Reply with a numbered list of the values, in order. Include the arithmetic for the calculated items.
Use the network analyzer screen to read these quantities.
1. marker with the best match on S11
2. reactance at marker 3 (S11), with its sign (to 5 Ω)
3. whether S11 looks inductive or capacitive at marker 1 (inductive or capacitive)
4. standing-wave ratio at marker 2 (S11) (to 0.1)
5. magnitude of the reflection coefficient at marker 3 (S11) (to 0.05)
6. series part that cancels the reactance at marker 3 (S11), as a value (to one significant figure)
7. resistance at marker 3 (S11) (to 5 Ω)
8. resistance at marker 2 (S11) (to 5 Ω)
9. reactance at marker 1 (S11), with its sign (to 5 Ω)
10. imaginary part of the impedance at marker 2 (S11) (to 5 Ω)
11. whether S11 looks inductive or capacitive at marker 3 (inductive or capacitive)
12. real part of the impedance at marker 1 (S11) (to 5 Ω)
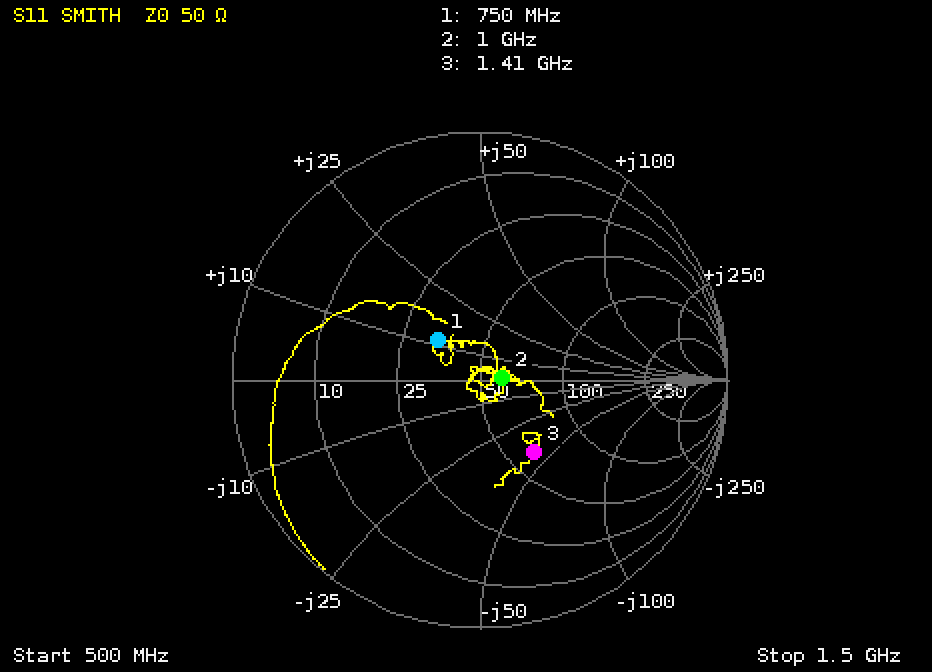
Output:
1. marker 2
2. -40 Ω
3. inductive
4. 1.2
5. 0.35
6. L = 40 Ω/(2π × 1.41 GHz) ≈ 5 nH
7. 60 Ω
8. 60 Ω
9. +10 Ω
10. 0 Ω
11. capacitive
12. 35 Ω
